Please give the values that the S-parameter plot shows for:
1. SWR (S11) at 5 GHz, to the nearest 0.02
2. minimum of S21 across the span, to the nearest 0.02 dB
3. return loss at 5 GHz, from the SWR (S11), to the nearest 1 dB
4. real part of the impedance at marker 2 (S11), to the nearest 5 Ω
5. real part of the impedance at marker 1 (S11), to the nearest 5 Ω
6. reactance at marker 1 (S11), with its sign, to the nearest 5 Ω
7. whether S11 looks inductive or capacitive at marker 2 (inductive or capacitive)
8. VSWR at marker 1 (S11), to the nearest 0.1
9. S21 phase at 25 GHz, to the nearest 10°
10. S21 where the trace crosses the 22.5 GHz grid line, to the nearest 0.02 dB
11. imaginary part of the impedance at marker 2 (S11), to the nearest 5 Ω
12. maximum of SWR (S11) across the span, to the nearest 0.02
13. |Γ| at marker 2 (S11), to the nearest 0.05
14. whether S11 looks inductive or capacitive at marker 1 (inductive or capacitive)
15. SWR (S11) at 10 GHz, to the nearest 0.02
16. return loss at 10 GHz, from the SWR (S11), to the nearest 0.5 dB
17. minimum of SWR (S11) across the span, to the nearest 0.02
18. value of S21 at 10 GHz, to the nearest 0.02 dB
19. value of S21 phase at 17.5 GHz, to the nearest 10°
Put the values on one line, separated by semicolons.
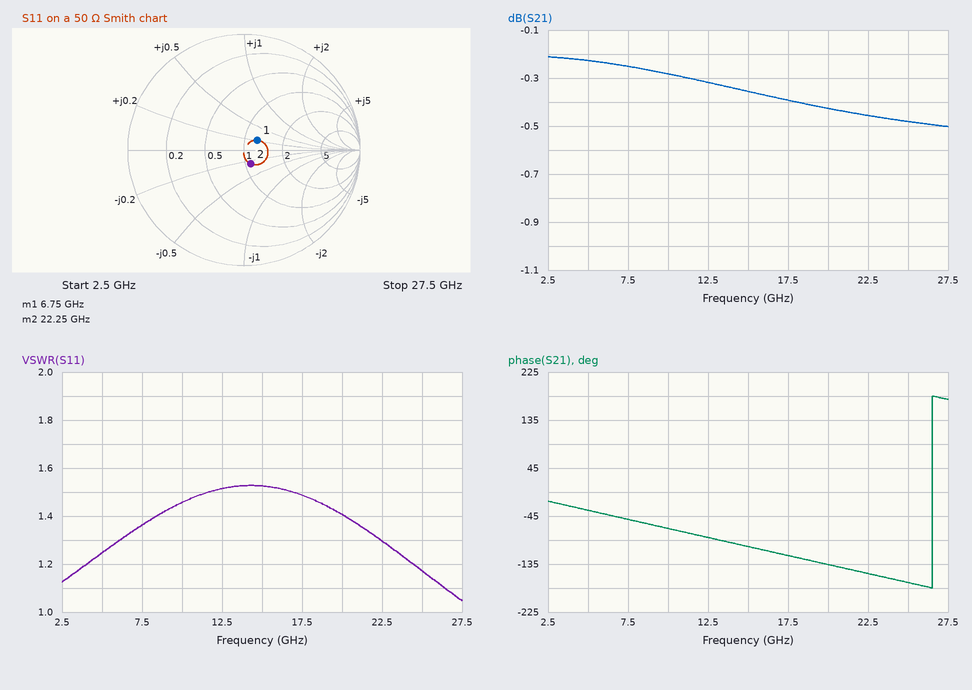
1.24; -0.50 dB; 19 dB; 55 Ω; 60 Ω; +10 Ω; capacitive; 1.3; -170°; -0.46 dB; -15 Ω; 1.52; 0.15; inductive; 1.46; 14.5 dB; 1.04; -0.28 dB; -120°
